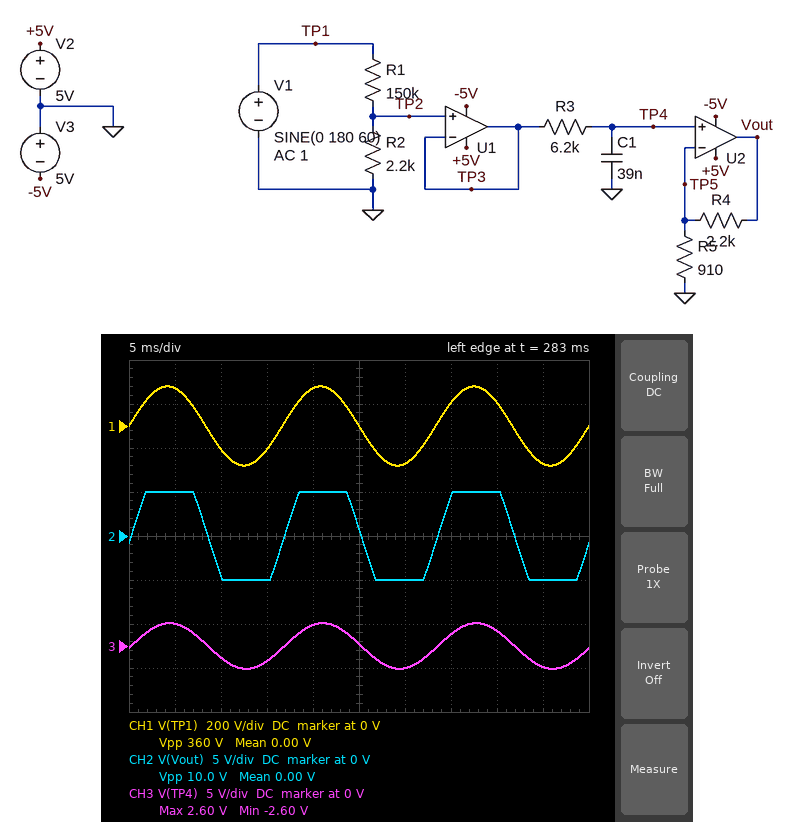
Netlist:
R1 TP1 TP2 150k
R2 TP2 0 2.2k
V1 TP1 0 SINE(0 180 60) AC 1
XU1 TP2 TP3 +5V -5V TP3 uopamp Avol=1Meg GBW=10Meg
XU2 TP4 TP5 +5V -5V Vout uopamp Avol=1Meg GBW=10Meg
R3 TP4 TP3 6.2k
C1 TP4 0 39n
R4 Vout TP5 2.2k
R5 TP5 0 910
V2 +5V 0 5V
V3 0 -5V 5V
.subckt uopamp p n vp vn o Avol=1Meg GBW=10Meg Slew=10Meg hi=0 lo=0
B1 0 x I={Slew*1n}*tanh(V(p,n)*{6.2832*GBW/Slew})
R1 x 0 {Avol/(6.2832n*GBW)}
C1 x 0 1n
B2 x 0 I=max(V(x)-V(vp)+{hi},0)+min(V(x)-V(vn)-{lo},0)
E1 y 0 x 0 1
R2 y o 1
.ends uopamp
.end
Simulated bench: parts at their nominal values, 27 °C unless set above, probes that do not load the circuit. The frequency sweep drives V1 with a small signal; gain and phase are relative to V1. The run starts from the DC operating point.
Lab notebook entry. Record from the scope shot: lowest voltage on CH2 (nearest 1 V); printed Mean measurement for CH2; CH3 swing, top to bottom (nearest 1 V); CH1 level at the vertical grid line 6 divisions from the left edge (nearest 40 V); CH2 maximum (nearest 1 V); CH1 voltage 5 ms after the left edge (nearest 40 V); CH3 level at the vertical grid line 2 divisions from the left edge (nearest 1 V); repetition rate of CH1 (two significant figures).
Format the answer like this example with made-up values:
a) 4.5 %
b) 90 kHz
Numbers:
a) -5 V
b) 0.00 V
c) 5 V
d) -160 V
e) 5 V
f) 160 V
g) -1 V
h) 60 Hz
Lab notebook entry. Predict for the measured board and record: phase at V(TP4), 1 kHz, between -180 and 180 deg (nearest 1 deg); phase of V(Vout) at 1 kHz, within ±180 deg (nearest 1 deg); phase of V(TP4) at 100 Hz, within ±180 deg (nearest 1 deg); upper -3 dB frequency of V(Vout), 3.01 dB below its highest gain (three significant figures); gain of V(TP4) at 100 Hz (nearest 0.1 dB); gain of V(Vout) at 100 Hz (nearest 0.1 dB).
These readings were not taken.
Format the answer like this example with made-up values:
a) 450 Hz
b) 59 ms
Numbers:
a) -57 deg
b) -57 deg
c) -9 deg
d) 658 Hz
e) -36.9 dB
f) -26.2 dB
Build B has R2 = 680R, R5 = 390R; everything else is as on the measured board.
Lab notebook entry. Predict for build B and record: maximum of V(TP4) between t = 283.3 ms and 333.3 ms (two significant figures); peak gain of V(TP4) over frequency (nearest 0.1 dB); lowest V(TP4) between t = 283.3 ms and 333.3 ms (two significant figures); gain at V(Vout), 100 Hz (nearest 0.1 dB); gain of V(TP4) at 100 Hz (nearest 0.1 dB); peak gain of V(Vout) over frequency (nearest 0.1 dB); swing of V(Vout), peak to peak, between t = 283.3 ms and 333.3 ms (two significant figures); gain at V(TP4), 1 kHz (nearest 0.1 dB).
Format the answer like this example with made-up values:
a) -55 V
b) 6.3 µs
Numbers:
a) 810 mV
b) -46.9 dB
c) -810 mV
d) -30.6 dB
e) -47.0 dB
f) -30.5 dB
g) 10 V
h) -52.1 dB
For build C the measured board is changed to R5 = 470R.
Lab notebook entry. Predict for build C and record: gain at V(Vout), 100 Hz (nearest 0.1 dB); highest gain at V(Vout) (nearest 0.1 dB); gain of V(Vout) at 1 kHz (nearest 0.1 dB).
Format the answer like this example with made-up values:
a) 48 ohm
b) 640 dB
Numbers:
a) -21.8 dB
b) -21.7 dB
c) -26.9 dB
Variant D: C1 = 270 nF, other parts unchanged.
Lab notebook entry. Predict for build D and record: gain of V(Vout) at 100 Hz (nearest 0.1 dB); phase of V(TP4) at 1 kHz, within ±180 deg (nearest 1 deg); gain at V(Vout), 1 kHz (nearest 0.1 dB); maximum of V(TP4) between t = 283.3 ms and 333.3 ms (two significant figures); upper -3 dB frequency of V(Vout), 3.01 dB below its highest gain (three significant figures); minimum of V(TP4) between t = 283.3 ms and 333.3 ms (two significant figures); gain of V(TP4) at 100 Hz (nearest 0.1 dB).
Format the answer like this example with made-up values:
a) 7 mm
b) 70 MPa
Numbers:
a) -29.4 dB
b) -85 deg
c) -46.6 dB
d) 2.2 V
e) 95.1 Hz
f) -2.2 V
g) -40.0 dB
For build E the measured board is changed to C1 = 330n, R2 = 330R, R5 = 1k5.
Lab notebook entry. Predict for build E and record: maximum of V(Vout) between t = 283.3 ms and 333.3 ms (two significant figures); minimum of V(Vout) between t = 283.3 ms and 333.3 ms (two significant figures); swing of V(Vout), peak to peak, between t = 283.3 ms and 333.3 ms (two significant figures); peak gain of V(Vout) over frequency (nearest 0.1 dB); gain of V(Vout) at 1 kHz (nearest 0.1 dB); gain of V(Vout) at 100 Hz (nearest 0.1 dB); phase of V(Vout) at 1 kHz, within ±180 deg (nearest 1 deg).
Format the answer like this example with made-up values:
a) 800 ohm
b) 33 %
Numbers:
a) 770 mV
b) -770 mV
c) 1.5 V
d) -45.3 dB
e) -67.5 dB
f) -49.6 dB
g) -86 deg
